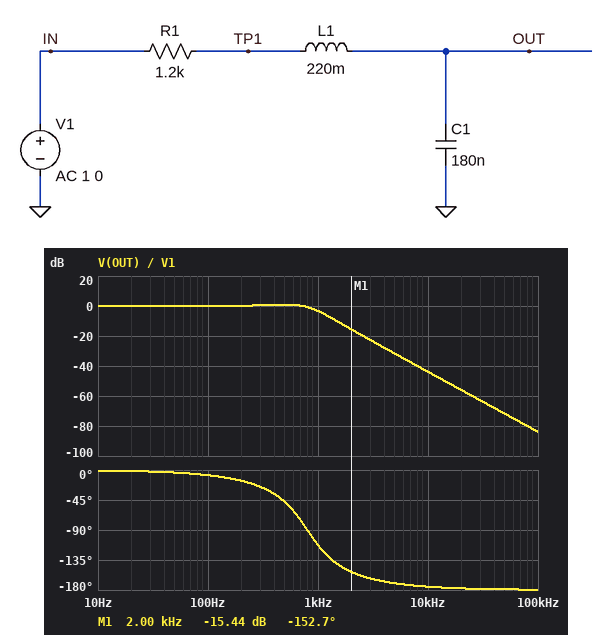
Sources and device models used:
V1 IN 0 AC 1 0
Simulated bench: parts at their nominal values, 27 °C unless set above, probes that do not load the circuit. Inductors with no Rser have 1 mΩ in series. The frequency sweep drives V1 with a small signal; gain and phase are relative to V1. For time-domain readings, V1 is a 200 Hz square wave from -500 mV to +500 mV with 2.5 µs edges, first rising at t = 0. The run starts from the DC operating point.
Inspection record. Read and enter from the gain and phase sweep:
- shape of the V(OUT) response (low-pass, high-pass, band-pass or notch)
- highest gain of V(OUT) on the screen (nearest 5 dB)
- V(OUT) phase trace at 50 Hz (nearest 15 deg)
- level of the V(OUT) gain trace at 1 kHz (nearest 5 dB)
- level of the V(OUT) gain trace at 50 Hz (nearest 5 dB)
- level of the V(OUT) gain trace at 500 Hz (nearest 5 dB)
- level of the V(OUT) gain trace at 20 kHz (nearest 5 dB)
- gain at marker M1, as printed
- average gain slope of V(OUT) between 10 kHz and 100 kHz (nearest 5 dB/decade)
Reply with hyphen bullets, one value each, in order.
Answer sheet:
- low-pass
- 0 dB
- 0 deg
- -5 dB
- 0 dB
- 0 dB
- -55 dB
- -15.44 dB
- -40 dB/decade
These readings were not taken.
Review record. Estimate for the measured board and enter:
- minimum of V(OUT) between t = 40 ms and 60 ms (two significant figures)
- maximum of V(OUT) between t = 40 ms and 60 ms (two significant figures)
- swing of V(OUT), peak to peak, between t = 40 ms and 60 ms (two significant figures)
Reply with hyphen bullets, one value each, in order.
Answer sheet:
- -630 mV
- 630 mV
- 1.3 V
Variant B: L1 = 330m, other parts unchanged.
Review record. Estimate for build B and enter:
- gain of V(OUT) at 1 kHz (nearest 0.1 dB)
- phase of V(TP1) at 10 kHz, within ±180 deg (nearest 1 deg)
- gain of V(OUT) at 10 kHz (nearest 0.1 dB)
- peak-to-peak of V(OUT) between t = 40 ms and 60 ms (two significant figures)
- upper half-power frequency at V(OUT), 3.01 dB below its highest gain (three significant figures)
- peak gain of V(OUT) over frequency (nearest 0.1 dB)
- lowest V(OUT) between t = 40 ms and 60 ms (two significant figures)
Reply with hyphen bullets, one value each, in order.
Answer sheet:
- -5.6 dB
- 3 deg
- -47.4 dB
- 1.4 V
- 773 Hz
- 2.0 dB
- -710 mV
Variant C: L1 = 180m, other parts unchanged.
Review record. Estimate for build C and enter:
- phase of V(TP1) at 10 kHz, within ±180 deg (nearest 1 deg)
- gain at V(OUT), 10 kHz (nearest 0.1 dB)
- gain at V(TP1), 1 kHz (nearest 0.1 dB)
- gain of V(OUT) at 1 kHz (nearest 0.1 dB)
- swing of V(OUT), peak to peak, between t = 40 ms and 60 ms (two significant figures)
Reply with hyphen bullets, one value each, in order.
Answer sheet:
- 6 deg
- -42.1 dB
- -13.9 dB
- -2.8 dB
- 1.2 V
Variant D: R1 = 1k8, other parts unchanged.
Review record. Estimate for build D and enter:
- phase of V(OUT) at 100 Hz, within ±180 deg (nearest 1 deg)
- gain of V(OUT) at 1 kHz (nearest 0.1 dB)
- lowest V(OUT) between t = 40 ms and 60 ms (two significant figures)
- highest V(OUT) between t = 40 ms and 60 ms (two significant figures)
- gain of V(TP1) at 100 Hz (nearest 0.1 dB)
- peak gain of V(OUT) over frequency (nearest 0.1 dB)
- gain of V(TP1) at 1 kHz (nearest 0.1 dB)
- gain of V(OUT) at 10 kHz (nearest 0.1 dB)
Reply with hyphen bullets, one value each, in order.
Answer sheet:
- -12 deg
- -6.5 dB
- -510 mV
- 510 mV
- -0.2 dB
- 0 dB
- -11.5 dB
- -43.9 dB
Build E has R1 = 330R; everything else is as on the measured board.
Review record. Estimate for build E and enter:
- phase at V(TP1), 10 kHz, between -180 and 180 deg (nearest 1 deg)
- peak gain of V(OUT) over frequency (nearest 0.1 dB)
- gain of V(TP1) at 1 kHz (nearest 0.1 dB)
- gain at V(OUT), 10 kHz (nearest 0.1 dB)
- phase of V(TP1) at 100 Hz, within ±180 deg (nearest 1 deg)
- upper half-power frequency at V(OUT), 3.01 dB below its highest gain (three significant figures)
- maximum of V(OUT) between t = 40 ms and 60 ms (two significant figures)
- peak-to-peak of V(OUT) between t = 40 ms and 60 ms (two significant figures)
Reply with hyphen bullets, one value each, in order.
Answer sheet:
- 1 deg
- 10.6 dB
- -1.6 dB
- -43.8 dB
- -2 deg
- 894 Hz
- 1.0 V
- 2.1 V
